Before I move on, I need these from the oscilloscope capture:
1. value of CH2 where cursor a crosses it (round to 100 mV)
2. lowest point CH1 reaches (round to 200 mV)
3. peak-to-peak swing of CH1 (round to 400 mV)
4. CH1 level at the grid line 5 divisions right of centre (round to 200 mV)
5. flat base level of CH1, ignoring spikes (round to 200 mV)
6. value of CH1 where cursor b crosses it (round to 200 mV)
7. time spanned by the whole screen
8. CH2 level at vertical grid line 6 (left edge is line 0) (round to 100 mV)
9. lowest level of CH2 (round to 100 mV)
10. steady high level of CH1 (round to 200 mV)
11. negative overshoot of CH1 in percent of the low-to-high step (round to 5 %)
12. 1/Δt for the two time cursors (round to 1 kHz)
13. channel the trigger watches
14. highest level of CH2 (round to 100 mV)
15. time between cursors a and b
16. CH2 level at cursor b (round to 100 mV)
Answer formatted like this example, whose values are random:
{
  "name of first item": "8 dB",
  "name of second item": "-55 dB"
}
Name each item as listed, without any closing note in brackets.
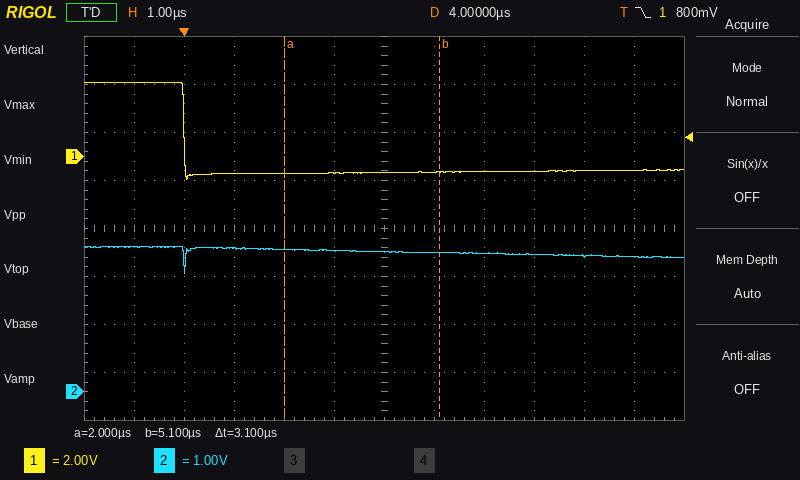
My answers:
{
  "value of CH2 where cursor a crosses it": "3.0 V",
  "lowest point CH1 reaches": "-1.0 V",
  "peak-to-peak swing of CH1": "4.0 V",
  "CH1 level at the grid line 5 divisions right of centre": "-600 mV",
  "flat base level of CH1, ignoring spikes": "-600 mV",
  "value of CH1 where cursor b crosses it": "-600 mV",
  "time spanned by the whole screen": "12 µs",
  "CH2 level at vertical grid line 6 (left edge is line 0)": "2.9 V",
  "lowest level of CH2": "2.5 V",
  "steady high level of CH1": "3.0 V",
  "negative overshoot of CH1 in percent of the low-to-high step": "10 %",
  "1/Δt for the two time cursors": "323 kHz",
  "channel the trigger watches": "CH1",
  "highest level of CH2": "3.0 V",
  "time between cursors a and b": "3.1 µs",
  "CH2 level at cursor b": "2.9 V"
}
